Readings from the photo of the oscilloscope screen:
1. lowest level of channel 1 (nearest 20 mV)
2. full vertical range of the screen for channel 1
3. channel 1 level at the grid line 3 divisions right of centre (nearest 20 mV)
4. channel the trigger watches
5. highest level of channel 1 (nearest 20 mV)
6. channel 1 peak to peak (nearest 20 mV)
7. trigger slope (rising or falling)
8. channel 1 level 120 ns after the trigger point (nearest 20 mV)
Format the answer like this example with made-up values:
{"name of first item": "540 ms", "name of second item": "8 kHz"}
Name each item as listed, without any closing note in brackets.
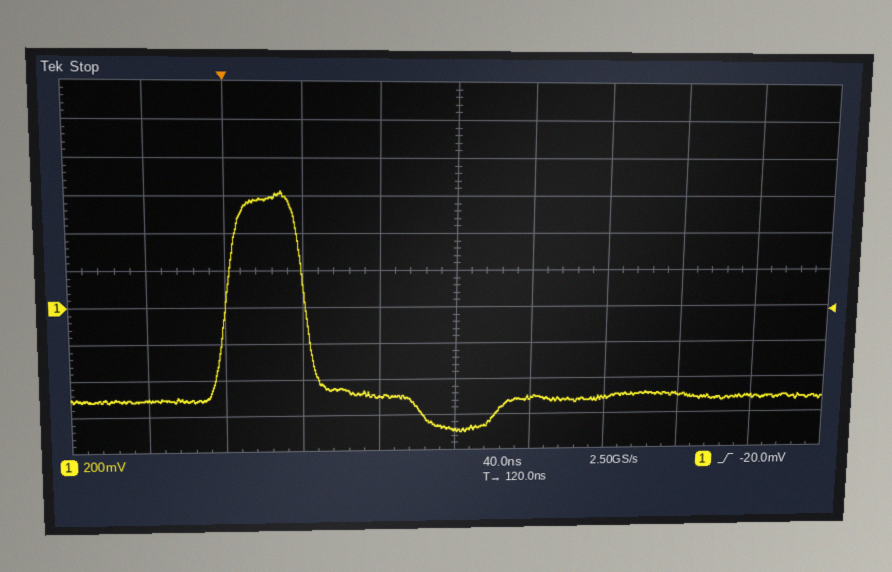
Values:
{"lowest level of channel 1": "-700 mV", "full vertical range of the screen for channel 1": "2 V", "channel 1 level at the grid line 3 divisions right of centre": "-500 mV", "channel the trigger watches": "channel 1", "highest level of channel 1": "620 mV", "channel 1 peak to peak": "1.32 V", "trigger slope": "rising", "channel 1 level 120 ns after the trigger point": "-680 mV"}
